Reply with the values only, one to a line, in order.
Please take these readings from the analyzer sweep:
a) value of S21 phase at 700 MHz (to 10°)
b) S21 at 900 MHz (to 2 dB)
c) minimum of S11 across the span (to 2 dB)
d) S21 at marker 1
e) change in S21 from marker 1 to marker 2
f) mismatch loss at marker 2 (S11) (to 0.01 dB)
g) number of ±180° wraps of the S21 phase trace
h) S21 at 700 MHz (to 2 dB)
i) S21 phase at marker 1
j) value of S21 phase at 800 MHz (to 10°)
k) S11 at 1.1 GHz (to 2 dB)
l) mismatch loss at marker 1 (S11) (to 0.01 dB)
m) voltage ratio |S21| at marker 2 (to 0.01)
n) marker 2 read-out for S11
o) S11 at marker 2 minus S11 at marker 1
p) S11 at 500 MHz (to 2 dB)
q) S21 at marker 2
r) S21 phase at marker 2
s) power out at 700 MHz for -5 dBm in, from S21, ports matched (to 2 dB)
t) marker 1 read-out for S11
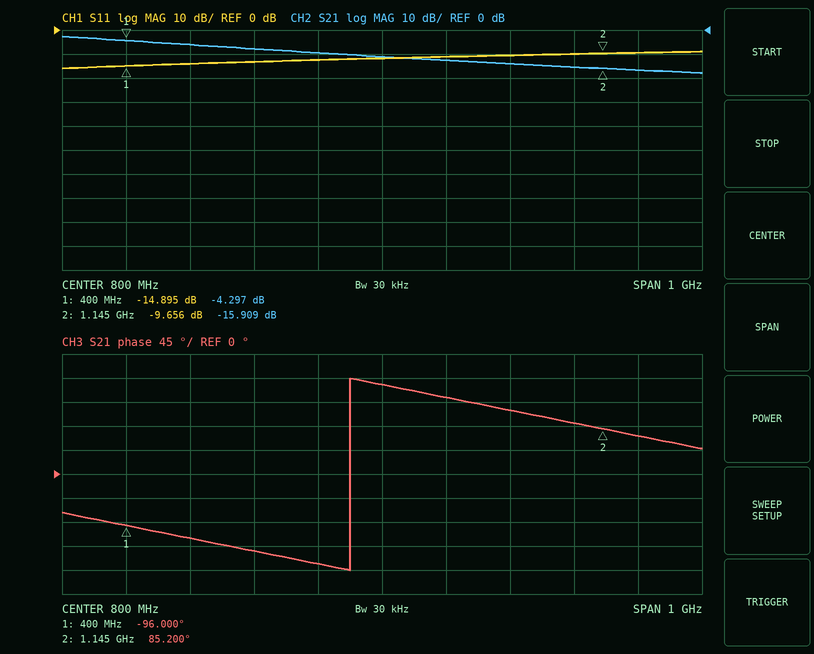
-170°
-12 dB
-16 dB
-4.297 dB
-11.612 dB
0.50 dB
1
-10 dB
-96.000°
170°
-10 dB
0.14 dB
0.16
-9.656 dB
5.239 dB
-14 dB
-15.909 dB
85.200°
-14 dBm
-14.895 dB
